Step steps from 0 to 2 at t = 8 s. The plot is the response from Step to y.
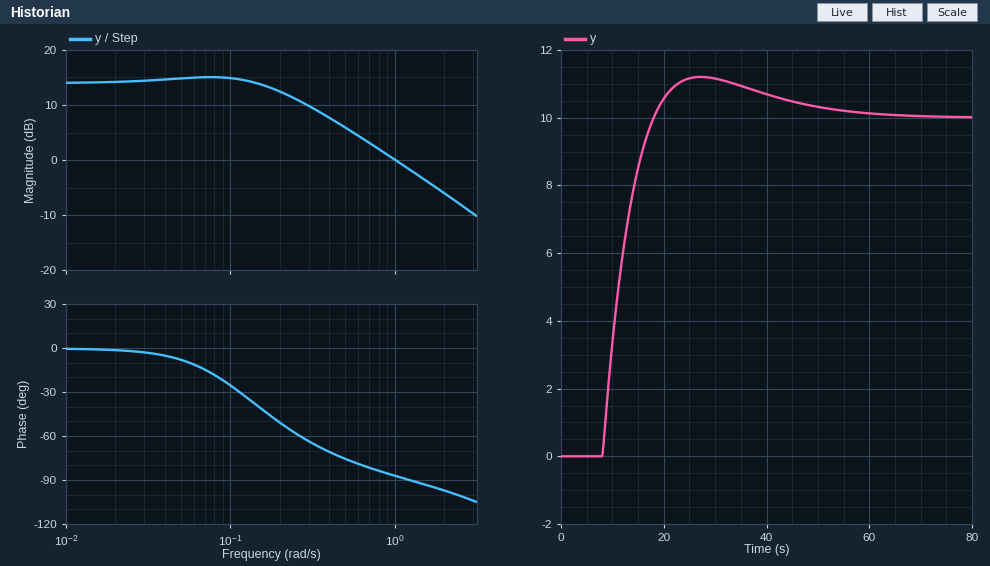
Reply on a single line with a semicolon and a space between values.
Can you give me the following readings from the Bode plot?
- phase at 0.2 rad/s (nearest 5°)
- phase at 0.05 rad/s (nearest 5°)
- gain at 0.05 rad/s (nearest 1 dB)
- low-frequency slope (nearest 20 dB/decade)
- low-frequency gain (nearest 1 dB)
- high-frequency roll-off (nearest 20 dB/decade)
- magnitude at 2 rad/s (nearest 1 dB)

-50°; -10°; 15 dB; 0 dB/decade; 14 dB; -20 dB/decade; -6 dB
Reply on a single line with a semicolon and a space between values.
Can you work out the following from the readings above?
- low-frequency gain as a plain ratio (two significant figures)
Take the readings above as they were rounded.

5.0
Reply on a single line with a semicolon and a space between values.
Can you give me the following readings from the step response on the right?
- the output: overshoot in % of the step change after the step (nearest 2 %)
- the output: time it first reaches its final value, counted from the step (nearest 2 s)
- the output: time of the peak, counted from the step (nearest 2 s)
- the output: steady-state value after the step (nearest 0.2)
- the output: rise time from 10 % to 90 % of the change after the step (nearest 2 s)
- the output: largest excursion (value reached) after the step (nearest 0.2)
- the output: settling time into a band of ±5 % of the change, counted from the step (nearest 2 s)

12 %; 10 s; 20 s; 10.0; 8 s; 11.2; 36 s
